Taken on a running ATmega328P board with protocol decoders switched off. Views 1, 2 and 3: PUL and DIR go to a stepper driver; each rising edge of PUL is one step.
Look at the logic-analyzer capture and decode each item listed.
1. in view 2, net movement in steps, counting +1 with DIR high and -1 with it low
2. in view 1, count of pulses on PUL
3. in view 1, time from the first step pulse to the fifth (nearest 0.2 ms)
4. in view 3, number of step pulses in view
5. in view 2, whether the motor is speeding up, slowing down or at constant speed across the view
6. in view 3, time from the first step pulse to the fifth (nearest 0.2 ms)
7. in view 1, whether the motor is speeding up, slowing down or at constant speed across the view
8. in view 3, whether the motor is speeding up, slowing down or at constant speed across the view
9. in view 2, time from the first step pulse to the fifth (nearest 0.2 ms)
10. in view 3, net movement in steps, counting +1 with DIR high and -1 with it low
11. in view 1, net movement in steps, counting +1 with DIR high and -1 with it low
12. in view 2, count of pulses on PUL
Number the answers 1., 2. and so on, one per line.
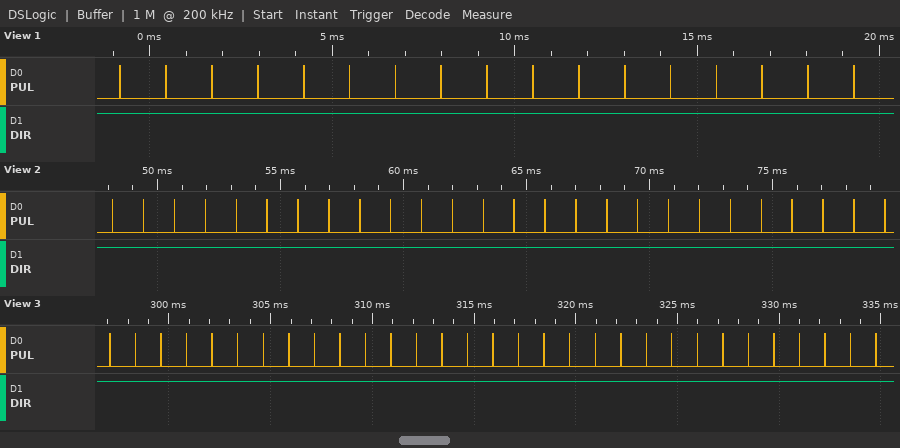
1. +26
2. 17
3. 5.0 ms
4. 31
5. constant speed
6. 5.0 ms
7. constant speed
8. constant speed
9. 5.0 ms
10. +31
11. +17
12. 26
